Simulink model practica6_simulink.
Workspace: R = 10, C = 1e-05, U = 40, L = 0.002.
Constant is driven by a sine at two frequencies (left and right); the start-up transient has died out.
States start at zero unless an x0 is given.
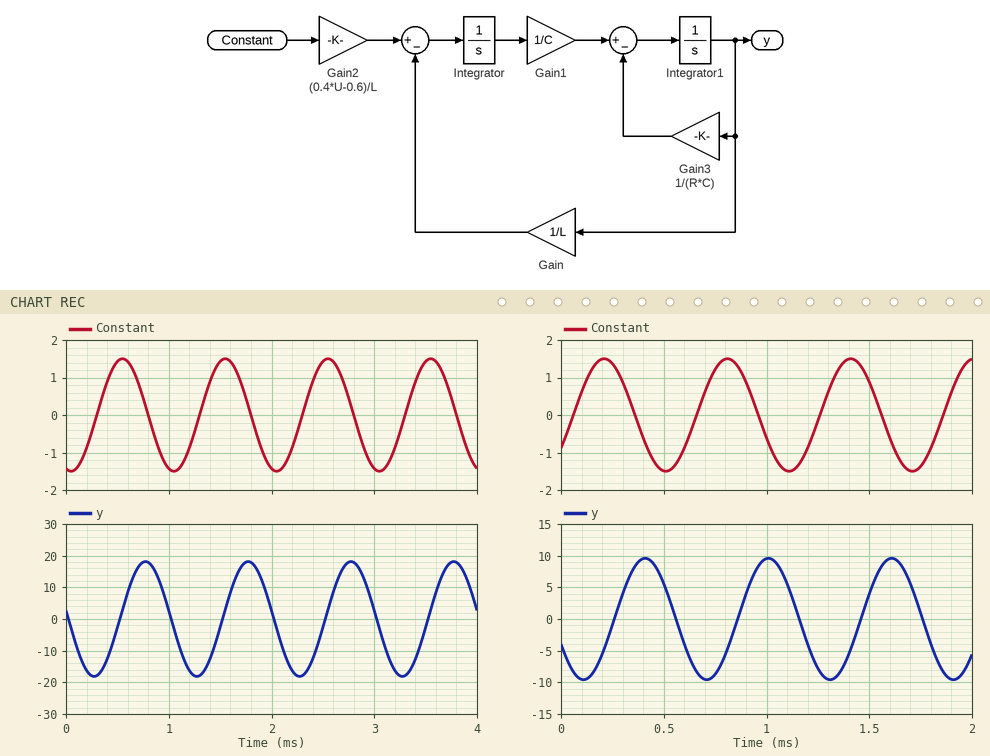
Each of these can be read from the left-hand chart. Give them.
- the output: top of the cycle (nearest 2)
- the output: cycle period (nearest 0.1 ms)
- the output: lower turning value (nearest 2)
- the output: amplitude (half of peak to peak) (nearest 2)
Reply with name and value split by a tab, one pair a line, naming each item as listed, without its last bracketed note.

the output: top of the cycle	18
the output: cycle period	1.0 ms
the output: lower turning value	-18
the output: amplitude (half of peak to peak)	18
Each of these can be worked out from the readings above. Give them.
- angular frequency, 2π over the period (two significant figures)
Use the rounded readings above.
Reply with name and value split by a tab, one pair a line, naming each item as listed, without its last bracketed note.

angular frequency, 2π over the period	6.3 rad/ms
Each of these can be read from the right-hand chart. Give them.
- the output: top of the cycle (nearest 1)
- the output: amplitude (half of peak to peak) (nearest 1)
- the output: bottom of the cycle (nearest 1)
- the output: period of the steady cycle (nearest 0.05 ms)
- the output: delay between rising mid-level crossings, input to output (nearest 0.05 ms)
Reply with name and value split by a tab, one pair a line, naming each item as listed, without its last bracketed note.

the output: top of the cycle	10
the output: amplitude (half of peak to peak)	10
the output: bottom of the cycle	-10
the output: period of the steady cycle	0.60 ms
the output: delay between rising mid-level crossings, input to output	0.20 ms
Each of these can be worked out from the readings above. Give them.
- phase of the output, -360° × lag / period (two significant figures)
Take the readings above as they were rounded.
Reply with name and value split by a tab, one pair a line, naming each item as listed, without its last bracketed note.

phase of the output, -360° × lag / period	-120°
